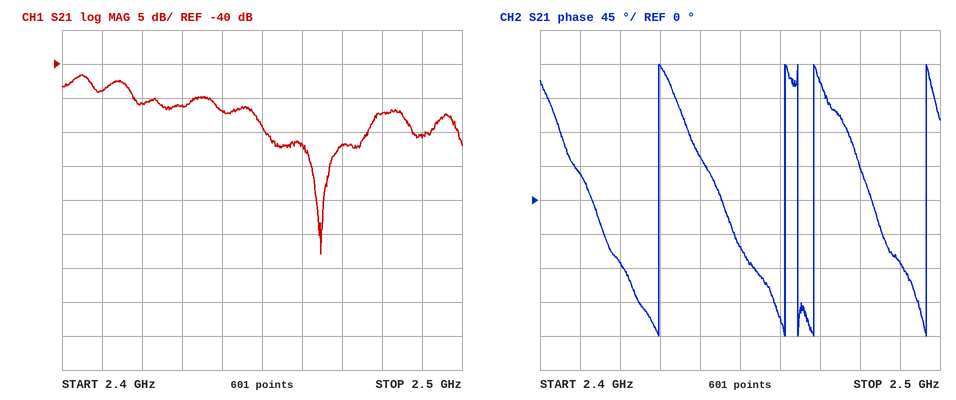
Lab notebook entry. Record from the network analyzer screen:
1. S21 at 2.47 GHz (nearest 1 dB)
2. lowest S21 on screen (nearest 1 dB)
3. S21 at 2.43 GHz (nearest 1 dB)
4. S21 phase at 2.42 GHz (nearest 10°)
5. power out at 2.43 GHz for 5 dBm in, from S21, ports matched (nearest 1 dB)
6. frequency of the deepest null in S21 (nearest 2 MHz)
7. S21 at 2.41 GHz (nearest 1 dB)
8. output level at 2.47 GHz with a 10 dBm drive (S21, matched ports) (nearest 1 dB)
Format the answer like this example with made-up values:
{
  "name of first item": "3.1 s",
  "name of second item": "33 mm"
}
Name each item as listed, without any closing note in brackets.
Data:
{
  "S21 at 2.47 GHz": "-52 dB",
  "lowest S21 on screen": "-68 dB",
  "S21 at 2.43 GHz": "-46 dB",
  "S21 phase at 2.42 GHz": "-80°",
  "power out at 2.43 GHz for 5 dBm in, from S21, ports matched": "-41 dBm",
  "frequency of the deepest null in S21": "2.464 GHz",
  "S21 at 2.41 GHz": "-44 dB",
  "output level at 2.47 GHz with a 10 dBm drive (S21, matched ports)": "-42 dBm"
}
